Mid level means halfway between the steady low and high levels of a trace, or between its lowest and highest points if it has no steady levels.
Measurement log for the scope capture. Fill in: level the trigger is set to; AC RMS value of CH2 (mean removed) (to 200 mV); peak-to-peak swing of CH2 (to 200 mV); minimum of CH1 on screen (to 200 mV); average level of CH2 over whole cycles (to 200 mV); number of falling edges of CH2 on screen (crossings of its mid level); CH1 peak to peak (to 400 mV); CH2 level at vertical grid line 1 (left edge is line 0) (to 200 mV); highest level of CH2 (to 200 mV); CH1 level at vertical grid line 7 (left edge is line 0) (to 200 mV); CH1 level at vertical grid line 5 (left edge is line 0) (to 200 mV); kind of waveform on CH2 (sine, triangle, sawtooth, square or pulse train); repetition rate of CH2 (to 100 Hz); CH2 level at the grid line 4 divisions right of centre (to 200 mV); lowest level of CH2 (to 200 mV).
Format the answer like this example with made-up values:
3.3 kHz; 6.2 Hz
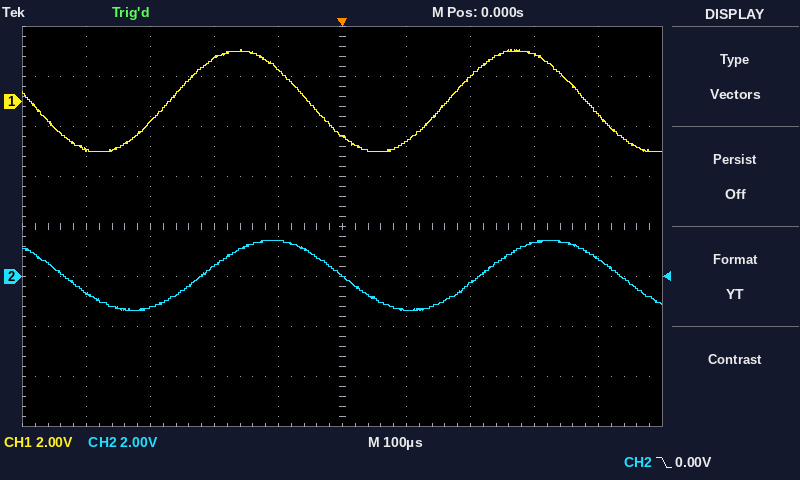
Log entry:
0.00 V; 1.0 V; 2.8 V; -2.0 V; 0.0 V; 3; 4.0 V; -600 mV; 1.4 V; 1.0 V; -1.4 V; sine; 2.3 kHz; 800 mV; -1.4 V
